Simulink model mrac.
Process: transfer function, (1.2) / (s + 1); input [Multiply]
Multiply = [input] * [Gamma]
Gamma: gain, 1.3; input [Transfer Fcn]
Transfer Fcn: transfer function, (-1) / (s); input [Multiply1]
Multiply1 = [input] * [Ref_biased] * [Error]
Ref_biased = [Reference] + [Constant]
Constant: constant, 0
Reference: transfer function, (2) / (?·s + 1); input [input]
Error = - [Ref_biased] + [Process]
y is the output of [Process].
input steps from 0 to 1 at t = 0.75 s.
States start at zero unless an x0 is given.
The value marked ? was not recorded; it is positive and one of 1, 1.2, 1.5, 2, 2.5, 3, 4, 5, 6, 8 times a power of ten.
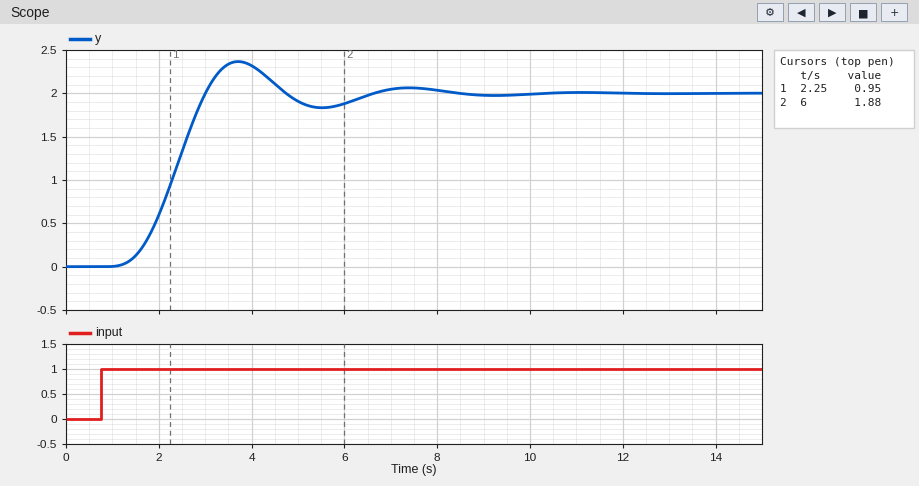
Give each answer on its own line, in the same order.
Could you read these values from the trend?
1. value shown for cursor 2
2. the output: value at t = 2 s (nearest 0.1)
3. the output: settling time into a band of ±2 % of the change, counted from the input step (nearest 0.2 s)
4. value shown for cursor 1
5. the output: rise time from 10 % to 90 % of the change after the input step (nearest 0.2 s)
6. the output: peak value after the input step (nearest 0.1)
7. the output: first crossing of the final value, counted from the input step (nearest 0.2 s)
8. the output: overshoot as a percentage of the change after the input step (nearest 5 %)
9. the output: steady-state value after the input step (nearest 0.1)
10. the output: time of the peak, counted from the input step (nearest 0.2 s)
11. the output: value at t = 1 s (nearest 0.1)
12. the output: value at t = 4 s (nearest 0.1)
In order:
1.88
0.6
7.2 s
0.95
1.2 s
2.4
2.2 s
20 %
2.0
3.0 s
0.0
2.3
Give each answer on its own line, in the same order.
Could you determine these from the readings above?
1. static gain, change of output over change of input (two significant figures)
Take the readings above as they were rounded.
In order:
2.0
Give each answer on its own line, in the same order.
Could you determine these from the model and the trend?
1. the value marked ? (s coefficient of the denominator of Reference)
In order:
0.8
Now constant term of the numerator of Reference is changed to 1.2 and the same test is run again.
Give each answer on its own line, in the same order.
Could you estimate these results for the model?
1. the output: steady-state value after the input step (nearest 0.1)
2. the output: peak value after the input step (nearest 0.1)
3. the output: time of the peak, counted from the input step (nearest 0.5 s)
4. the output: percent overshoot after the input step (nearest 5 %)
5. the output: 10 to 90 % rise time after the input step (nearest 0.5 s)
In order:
1.2
1.4
3.5 s
15 %
1.5 s
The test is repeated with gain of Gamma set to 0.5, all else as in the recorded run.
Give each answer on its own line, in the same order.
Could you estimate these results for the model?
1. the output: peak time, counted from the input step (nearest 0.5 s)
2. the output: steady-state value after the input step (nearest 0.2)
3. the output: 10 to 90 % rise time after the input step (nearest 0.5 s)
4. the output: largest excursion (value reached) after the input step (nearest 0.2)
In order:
4.5 s
2.0
2.0 s
2.2
